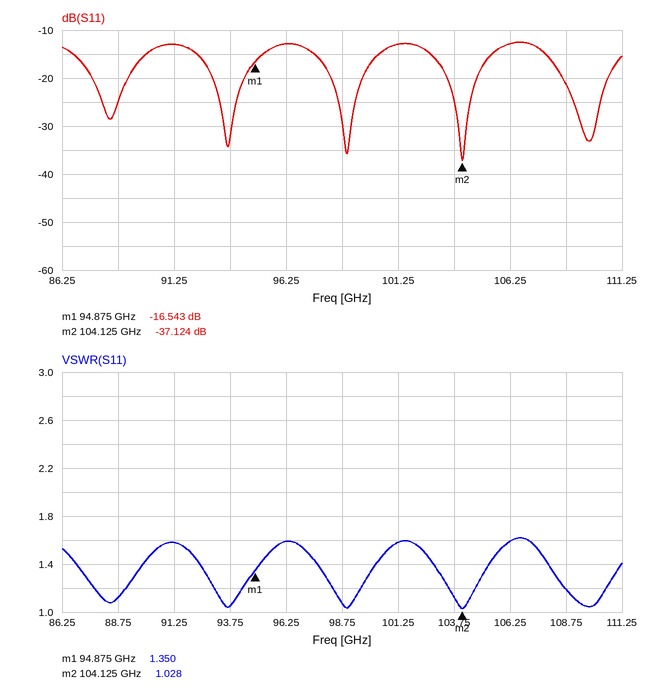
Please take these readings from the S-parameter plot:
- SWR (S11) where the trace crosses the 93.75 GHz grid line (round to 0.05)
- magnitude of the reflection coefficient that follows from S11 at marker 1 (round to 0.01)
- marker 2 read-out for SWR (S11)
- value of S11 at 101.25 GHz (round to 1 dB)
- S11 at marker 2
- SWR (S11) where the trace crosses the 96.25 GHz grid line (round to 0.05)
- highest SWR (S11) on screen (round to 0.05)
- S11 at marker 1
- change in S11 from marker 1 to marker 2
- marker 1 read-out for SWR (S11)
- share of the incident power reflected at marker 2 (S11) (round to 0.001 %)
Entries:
1.05
0.15
1.028
-13 dB
-37.124 dB
1.60
1.60
-16.543 dB
-20.581 dB
1.350
0.019 %
